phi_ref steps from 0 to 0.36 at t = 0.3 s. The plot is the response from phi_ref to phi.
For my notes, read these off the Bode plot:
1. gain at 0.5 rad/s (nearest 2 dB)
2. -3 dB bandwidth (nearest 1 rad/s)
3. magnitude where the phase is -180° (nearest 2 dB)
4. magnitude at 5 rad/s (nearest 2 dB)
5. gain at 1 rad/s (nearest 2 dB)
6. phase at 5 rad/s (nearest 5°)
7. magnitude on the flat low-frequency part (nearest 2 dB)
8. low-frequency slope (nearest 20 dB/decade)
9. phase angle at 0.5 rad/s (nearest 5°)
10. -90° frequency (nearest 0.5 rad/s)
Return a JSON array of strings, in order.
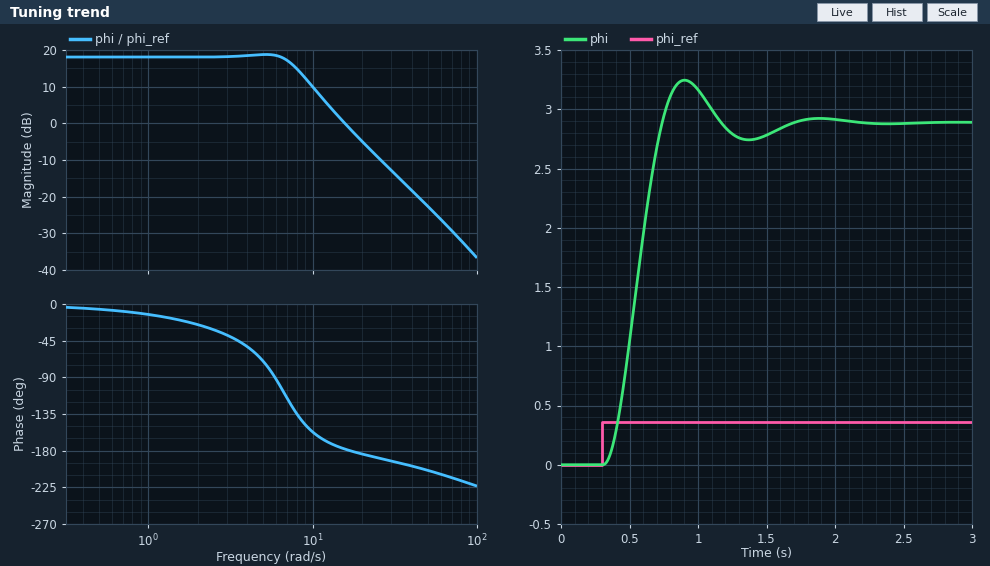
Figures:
["18 dB", "8 rad/s", "-2 dB", "18 dB", "18 dB", "-70°", "18 dB", "0 dB/decade", "-5°", "6.0 rad/s"]
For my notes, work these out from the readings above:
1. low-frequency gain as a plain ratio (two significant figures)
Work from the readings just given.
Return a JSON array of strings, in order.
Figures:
["7.9"]
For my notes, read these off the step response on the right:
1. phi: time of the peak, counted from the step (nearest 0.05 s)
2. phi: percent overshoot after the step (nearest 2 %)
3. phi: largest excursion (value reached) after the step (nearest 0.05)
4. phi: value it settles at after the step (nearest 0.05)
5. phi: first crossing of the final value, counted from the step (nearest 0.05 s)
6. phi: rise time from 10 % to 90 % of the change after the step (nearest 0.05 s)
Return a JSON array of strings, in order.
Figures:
["0.60 s", "12 %", "3.25", "2.90", "0.45 s", "0.30 s"]
